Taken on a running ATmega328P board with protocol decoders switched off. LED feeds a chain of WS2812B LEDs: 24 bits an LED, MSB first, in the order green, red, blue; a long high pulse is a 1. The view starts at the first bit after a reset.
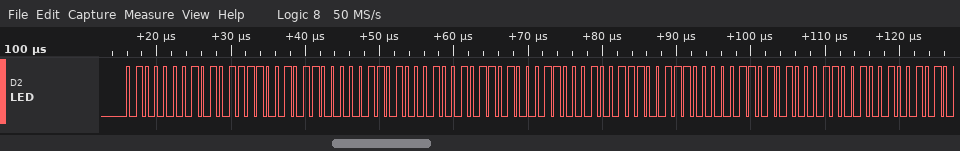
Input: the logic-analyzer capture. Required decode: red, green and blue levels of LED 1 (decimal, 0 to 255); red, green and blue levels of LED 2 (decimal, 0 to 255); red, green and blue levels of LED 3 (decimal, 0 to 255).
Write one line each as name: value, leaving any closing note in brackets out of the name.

red, green and blue levels of LED 1: 94, 65, 88
red, green and blue levels of LED 2: 75, 52, 70
red, green and blue levels of LED 3: 56, 39, 53
